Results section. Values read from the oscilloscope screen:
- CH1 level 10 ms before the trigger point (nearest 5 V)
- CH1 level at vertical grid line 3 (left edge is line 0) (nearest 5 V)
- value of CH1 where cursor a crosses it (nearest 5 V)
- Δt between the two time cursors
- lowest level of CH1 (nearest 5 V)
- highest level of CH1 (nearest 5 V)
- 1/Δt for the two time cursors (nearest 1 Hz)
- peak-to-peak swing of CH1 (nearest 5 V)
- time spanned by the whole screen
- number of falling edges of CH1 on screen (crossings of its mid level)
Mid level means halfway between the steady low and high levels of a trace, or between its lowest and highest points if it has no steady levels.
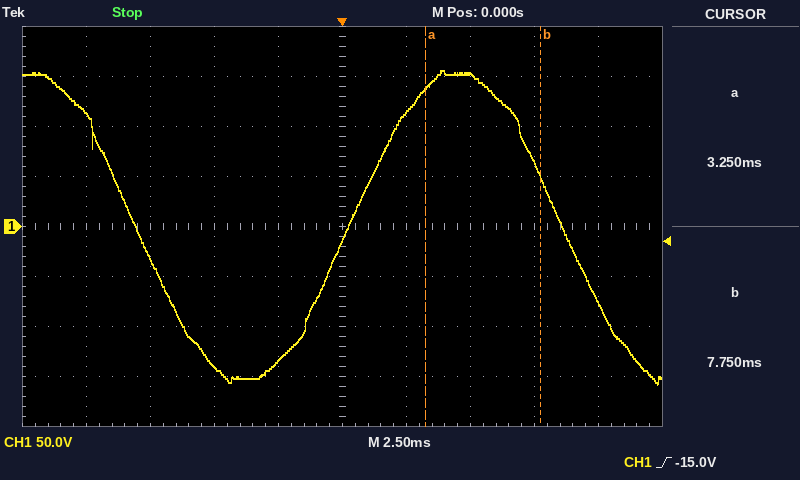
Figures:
115 V
-140 V
140 V
4.50 ms
-160 V
155 V
222 Hz
315 V
25 ms
2
